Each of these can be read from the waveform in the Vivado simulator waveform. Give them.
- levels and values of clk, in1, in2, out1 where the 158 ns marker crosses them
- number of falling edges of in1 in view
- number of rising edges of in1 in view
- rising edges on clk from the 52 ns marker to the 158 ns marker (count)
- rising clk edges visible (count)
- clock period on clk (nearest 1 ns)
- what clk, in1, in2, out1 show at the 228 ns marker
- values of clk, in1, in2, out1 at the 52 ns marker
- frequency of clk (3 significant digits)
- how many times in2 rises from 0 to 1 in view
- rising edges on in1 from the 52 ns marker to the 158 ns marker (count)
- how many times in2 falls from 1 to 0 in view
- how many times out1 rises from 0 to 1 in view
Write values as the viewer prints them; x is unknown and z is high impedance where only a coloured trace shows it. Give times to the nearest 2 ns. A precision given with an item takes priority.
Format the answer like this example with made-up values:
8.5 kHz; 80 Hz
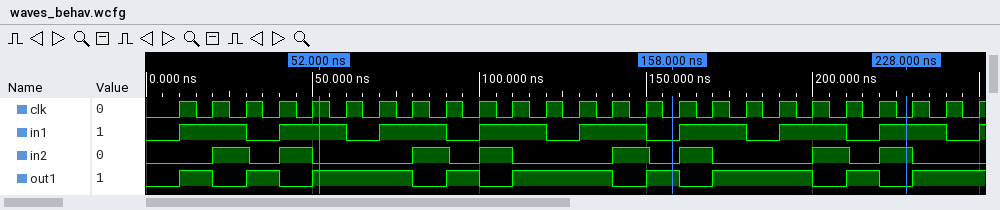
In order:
clk=0, in1=0, in2=0, out1=1; 8; 9; 10; 25; 10 ns; clk=0, in1=1, in2=1, out1=0; clk=1, in1=1, in2=0, out1=1; 100 MHz; 8; 3; 8; 9
